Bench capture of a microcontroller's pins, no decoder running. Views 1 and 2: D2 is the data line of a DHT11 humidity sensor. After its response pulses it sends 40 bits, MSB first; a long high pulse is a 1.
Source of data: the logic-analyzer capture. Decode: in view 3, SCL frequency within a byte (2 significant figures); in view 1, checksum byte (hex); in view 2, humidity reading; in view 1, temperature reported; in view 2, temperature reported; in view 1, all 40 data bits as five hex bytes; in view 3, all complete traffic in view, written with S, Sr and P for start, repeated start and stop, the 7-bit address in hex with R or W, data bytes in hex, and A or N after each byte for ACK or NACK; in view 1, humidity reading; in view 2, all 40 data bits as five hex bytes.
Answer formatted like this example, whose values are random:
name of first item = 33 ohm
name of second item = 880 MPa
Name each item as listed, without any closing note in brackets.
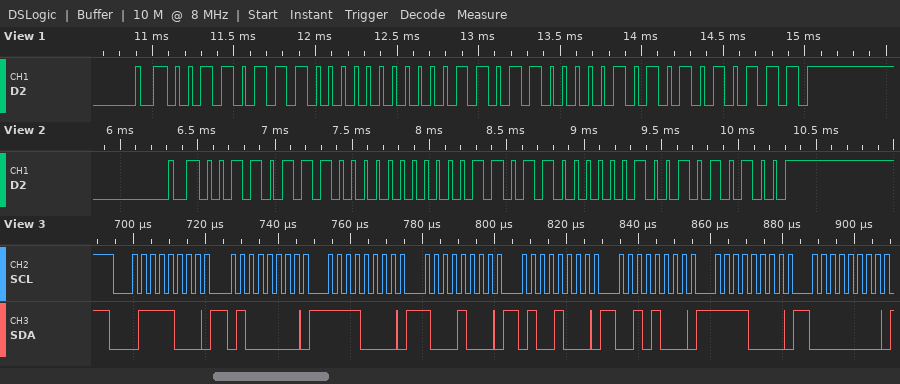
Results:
in view 3, SCL frequency within a byte = 400 kHz
in view 1, checksum byte = 0x57
in view 2, humidity reading = 55 %
in view 1, temperature reported = 27.5 °C
in view 2, temperature reported = 27.2 °C
in view 1, all 40 data bits as five hex bytes = 37 00 1B 05 57
in view 3, all complete traffic in view, written with S, Sr and P for start, repeated start and stop, the 7-bit address in hex with R or W, data bytes in hex, and A or N after each byte for ACK or NACK = S 3CW A 40 A F0 A 88 A 48 A 28 A F0 A 00 A
in view 1, humidity reading = 55 %
in view 2, all 40 data bits as five hex bytes = 37 00 1B 02 54
